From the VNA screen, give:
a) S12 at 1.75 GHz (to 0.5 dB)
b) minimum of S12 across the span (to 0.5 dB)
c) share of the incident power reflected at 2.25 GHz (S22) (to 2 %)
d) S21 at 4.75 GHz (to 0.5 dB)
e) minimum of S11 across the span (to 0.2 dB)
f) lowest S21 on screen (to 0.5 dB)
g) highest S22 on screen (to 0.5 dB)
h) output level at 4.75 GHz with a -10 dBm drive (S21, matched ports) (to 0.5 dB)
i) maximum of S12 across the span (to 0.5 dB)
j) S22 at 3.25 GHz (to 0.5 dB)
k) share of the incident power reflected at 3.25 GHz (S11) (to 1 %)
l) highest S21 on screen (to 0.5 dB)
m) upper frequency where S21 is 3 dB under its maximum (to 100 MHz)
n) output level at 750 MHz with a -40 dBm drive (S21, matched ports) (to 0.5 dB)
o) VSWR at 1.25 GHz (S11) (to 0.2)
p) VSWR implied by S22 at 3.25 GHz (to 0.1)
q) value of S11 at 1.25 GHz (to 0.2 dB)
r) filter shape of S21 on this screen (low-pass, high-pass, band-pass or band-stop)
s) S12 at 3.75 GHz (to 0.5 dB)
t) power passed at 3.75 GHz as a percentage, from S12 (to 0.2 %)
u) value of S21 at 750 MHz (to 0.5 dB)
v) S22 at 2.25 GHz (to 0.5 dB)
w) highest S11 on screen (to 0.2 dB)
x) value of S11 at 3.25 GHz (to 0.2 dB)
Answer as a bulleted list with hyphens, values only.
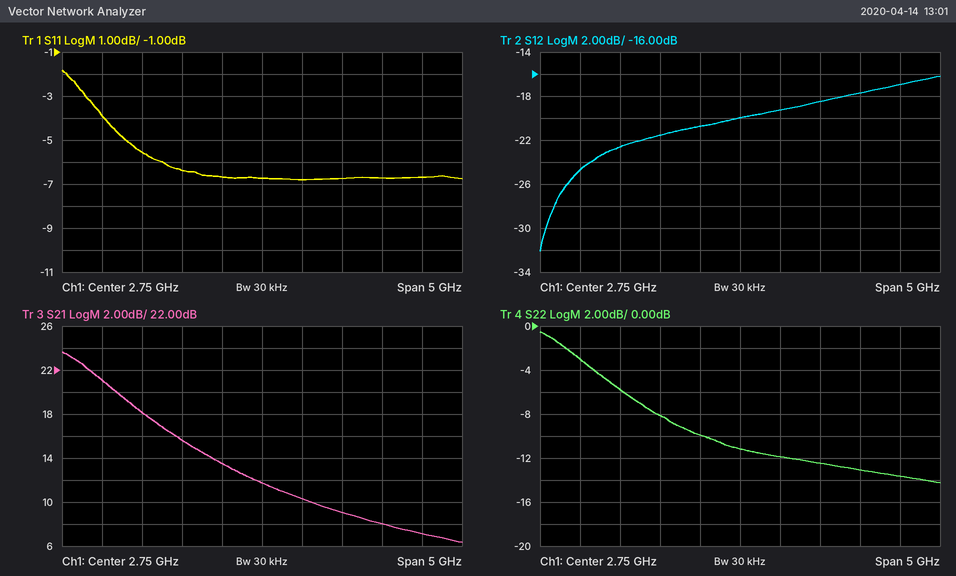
- -21.5 dB
- -32.0 dB
- 10 %
- 7.0 dB
- -6.8 dB
- 6.5 dB
- -0.5 dB
- -3.0 dBm
- -16.0 dB
- -12.0 dB
- 21 %
- 23.5 dB
- 800 MHz
- -19.0 dBm
- 3.2
- 1.7
- -5.6 dB
- low-pass
- -18.5 dB
- 1.4 %
- 21.0 dB
- -10.0 dB
- -1.8 dB
- -6.8 dB
